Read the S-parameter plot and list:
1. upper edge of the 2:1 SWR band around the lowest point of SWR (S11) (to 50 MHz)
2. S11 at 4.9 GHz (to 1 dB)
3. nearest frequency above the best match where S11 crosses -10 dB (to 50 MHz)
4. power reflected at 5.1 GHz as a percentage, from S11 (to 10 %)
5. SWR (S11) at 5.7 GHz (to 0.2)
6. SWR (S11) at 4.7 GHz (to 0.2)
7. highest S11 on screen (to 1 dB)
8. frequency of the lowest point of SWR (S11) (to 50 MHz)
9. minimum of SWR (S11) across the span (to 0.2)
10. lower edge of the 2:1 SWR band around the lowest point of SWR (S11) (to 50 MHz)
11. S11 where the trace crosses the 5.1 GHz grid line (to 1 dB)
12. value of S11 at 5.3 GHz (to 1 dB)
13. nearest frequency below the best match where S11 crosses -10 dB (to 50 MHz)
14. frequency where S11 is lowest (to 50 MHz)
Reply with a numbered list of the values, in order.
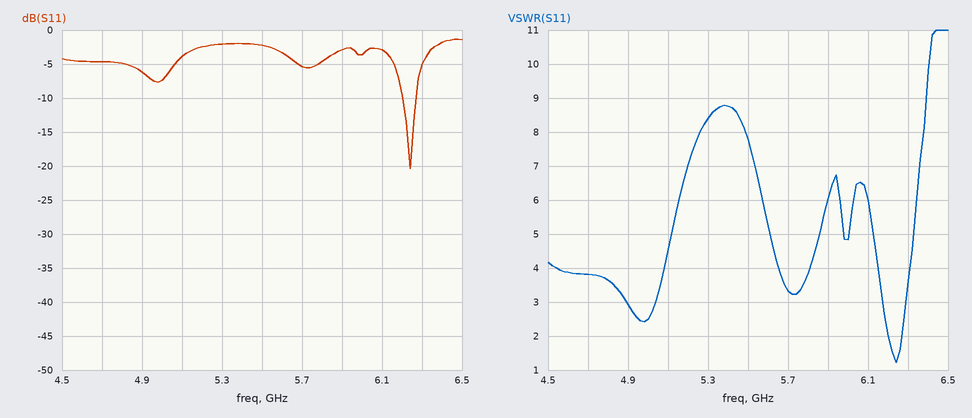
1. 6.25 GHz
2. -6 dB
3. 6.25 GHz
4. 40 %
5. 3.4
6. 3.8
7. -1 dB
8. 6.25 GHz
9. 1.2
10. 6.20 GHz
11. -4 dB
12. -2 dB
13. 6.20 GHz
14. 6.25 GHz
